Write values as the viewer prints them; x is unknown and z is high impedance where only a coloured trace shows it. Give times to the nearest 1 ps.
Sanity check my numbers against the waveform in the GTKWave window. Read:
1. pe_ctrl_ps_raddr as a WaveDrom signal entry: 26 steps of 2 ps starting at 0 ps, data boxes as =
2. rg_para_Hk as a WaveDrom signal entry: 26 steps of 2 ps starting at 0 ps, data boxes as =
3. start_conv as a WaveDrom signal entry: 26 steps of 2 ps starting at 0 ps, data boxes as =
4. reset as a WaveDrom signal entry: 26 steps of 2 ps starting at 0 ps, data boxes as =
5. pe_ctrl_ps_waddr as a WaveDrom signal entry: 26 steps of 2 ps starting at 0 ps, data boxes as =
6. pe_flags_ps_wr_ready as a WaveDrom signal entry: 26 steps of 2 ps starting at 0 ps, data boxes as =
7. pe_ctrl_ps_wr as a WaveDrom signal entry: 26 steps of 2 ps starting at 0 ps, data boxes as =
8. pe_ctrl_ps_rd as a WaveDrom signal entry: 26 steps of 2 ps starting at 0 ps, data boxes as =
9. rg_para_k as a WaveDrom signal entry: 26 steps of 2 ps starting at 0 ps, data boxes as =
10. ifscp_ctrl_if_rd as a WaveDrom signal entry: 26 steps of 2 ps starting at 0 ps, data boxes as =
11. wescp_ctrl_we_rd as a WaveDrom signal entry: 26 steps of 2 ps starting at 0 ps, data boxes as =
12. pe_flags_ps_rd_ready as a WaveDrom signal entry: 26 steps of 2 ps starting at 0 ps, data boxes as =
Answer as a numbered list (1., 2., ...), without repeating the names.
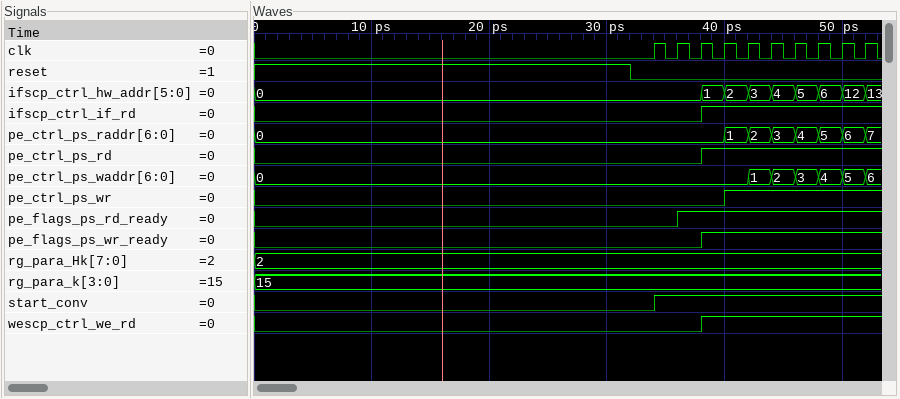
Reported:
1. {name: 'pe_ctrl_ps_raddr', wave: '=...................======', data: '0 1 2 3 4 5 6'}
2. {name: 'rg_para_Hk', wave: '=.........................', data: '2'}
3. {name: 'start_conv', wave: '0................1........'}
4. {name: 'reset', wave: '1...............0.........'}
5. {name: 'pe_ctrl_ps_waddr', wave: '=....................=====', data: '0 1 2 3 4 5'}
6. {name: 'pe_flags_ps_wr_ready', wave: '0..................1......'}
7. {name: 'pe_ctrl_ps_wr', wave: '0...................1.....'}
8. {name: 'pe_ctrl_ps_rd', wave: '0..................1......'}
9. {name: 'rg_para_k', wave: '=.........................', data: '15'}
10. {name: 'ifscp_ctrl_if_rd', wave: '0..................1......'}
11. {name: 'wescp_ctrl_we_rd', wave: '0..................1......'}
12. {name: 'pe_flags_ps_rd_ready', wave: '0.................1.......'}
